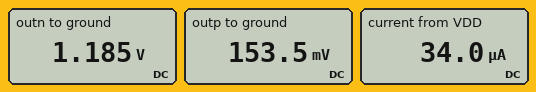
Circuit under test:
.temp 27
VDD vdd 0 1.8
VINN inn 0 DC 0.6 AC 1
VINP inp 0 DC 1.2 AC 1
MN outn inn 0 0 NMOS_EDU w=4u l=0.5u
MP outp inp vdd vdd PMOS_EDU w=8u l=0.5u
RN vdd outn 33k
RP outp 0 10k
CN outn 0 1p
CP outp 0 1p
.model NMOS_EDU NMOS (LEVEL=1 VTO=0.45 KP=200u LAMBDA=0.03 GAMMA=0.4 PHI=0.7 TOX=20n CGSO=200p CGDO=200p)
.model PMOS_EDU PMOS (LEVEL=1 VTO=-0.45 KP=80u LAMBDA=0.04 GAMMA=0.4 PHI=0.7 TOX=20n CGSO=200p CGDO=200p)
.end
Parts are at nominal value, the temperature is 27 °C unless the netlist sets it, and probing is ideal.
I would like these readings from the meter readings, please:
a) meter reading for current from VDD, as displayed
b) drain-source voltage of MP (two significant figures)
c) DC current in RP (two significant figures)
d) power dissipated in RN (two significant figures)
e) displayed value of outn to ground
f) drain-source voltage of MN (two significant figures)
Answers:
34.0 µA
-1.6 V
15 µA
11 µW
1.185 V
1.2 V
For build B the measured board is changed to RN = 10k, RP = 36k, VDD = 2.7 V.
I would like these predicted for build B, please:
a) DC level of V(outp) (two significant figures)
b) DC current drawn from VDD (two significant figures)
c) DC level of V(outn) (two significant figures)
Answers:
2.6 V
93 µA
2.5 V
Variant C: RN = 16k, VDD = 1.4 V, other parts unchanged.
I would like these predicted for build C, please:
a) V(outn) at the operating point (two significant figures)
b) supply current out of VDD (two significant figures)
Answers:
1.1 V
19 µA
